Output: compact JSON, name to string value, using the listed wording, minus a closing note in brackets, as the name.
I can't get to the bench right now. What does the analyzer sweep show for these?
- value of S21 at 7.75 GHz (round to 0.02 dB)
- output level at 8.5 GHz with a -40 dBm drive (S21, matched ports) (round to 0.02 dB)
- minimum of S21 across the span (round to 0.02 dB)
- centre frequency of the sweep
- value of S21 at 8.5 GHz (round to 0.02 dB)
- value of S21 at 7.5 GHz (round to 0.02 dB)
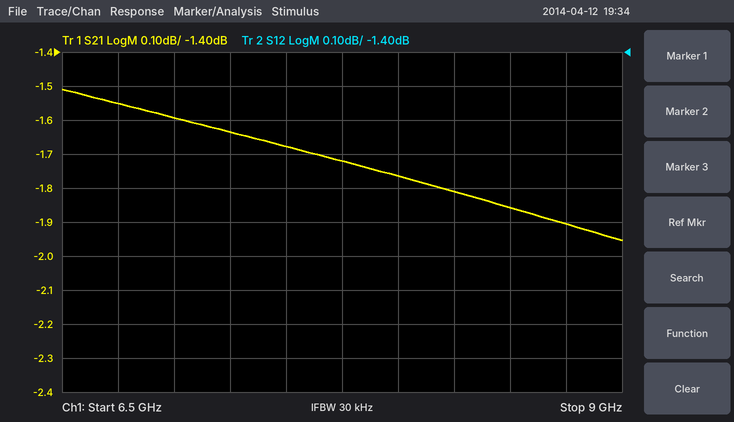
{"value of S21 at 7.75 GHz": "-1.72 dB", "output level at 8.5 GHz with a -40 dBm drive (S21, matched ports)": "-41.86 dBm", "minimum of S21 across the span": "-1.96 dB", "centre frequency of the sweep": "7.75 GHz", "value of S21 at 8.5 GHz": "-1.86 dB", "value of S21 at 7.5 GHz": "-1.68 dB"}
